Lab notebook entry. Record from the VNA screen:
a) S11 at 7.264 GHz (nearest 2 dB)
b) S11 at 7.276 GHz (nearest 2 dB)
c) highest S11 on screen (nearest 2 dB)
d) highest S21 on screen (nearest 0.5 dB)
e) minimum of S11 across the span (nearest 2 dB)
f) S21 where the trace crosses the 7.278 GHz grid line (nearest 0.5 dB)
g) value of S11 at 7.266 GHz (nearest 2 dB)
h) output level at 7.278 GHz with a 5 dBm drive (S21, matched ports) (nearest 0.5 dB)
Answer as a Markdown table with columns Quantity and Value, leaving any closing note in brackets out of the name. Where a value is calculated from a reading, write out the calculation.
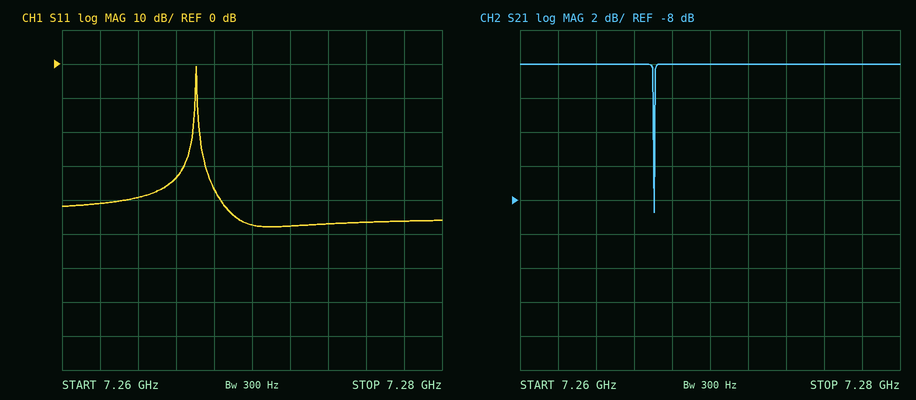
| Quantity | Value |
|---|---|
| S11 at 7.264 GHz | -40 dB |
| S11 at 7.276 GHz | -46 dB |
| highest S11 on screen | 0 dB |
| highest S21 on screen | 0.0 dB |
| minimum of S11 across the span | -48 dB |
| S21 where the trace crosses the 7.278 GHz grid line | 0.0 dB |
| value of S11 at 7.266 GHz | -34 dB |
| output level at 7.278 GHz with a 5 dBm drive (S21, matched ports) | 5 dBm + (0.0 dB) = 5.0 dBm |
